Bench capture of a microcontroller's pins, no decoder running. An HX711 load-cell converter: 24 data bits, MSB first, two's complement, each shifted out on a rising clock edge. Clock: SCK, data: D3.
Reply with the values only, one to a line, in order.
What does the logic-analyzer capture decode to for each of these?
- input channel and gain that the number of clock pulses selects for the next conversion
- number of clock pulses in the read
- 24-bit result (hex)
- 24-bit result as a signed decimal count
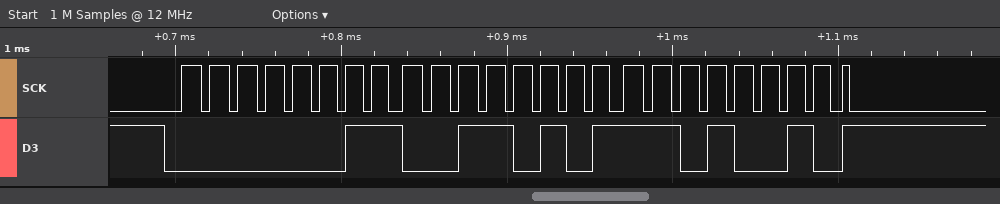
channel A, gain 128
25
0x0335D2
210386
